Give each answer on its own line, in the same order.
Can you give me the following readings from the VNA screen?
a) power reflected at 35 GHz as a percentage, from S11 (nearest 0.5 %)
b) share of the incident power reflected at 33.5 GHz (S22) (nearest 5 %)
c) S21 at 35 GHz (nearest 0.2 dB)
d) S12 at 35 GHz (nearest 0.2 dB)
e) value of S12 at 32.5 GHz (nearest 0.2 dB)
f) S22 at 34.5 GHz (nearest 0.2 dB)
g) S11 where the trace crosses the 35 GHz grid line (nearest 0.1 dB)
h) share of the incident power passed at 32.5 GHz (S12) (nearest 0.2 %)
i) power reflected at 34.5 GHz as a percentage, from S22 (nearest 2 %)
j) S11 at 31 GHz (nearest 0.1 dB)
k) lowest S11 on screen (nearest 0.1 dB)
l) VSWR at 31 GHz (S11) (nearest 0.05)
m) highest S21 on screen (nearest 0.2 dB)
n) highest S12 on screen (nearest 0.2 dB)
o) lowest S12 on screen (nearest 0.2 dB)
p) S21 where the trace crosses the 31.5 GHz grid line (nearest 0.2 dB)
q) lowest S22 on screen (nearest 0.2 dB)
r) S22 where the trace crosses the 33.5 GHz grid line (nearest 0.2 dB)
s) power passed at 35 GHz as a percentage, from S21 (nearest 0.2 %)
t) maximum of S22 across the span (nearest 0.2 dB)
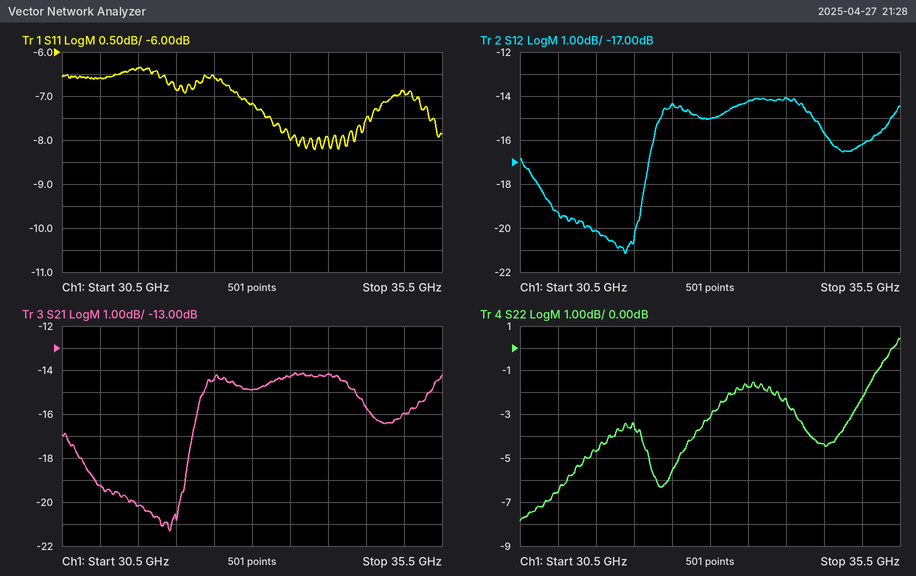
20.5 %
65 %
-16.0 dB
-16.2 dB
-14.4 dB
-4.4 dB
-6.9 dB
3.6 %
36 %
-6.6 dB
-8.2 dB
2.75
-14.2 dB
-14.0 dB
-21.2 dB
-20.2 dB
-7.8 dB
-1.8 dB
2.6 %
0.4 dB
